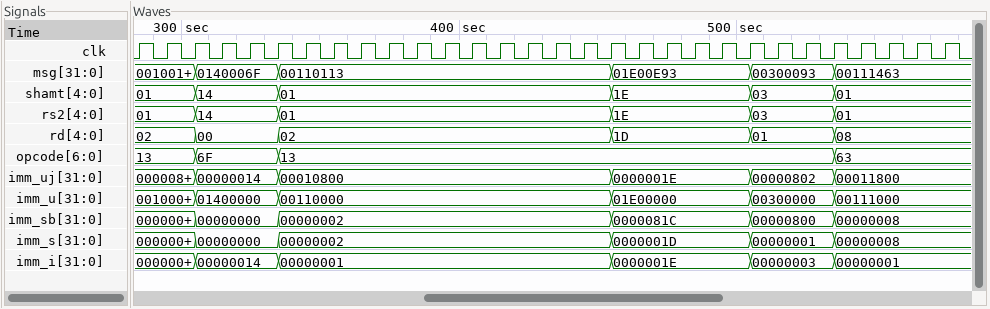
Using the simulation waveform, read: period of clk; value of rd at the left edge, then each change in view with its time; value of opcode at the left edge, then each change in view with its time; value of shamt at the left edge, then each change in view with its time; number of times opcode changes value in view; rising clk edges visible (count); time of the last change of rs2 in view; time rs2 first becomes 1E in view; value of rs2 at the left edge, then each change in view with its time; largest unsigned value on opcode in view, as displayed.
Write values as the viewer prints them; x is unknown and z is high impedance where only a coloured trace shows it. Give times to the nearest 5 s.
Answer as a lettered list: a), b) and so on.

a) 10 s
b) 02, 00 at 305 s, 02 at 335 s, 1D at 455 s, 01 at 505 s, 08 at 535 s
c) 13, 6F at 305 s, 13 at 335 s, 63 at 535 s
d) 01, 14 at 305 s, 01 at 335 s, 1E at 455 s, 03 at 505 s, 01 at 535 s
e) 3
f) 30
g) 535 s
h) 455 s
i) 01, 14 at 305 s, 01 at 335 s, 1E at 455 s, 03 at 505 s, 01 at 535 s
j) 6F
